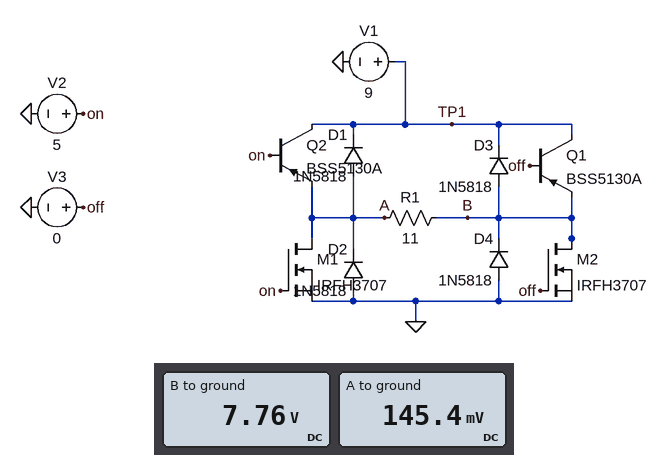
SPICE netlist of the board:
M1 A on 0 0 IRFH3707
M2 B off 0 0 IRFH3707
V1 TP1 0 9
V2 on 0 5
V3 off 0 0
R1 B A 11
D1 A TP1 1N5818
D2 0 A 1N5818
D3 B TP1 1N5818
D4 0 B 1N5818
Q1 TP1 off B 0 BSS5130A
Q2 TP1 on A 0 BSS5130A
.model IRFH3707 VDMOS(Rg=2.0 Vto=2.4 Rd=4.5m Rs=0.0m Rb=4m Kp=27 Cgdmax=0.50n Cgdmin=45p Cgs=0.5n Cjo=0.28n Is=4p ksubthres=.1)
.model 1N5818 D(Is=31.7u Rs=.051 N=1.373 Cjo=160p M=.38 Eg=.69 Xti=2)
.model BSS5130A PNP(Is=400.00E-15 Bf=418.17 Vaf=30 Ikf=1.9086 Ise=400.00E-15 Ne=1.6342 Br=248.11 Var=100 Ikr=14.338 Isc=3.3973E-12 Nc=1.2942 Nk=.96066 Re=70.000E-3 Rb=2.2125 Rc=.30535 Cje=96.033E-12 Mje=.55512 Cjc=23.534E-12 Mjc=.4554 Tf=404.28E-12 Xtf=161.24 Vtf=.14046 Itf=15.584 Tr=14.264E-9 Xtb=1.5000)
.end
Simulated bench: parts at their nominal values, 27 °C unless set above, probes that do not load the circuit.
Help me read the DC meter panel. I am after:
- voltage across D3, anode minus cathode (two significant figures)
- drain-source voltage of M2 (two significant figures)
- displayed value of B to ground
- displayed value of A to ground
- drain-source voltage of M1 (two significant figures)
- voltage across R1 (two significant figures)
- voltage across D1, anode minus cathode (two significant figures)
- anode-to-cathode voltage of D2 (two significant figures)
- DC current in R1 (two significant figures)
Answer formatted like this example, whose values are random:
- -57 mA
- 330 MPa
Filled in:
- -1.2 V
- 7.8 V
- 7.76 V
- 145.4 mV
- 150 mV
- 7.6 V
- -8.9 V
- -150 mV
- 690 mA
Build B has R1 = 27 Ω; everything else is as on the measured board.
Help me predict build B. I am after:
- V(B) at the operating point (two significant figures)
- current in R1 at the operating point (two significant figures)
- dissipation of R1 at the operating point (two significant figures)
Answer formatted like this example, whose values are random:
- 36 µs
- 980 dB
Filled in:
- 7.9 V
- 290 mA
- 2.2 W
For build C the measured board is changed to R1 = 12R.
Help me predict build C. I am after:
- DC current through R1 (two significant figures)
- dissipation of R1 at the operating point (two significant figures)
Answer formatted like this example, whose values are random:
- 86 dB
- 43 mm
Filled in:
- 640 mA
- 4.9 W
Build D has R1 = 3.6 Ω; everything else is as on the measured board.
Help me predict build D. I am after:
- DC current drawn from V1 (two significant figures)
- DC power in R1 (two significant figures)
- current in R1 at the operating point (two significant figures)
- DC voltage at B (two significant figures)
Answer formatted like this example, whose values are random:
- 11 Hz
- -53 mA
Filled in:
- 12 A
- 14 W
- 2.0 A
- 7.3 V
